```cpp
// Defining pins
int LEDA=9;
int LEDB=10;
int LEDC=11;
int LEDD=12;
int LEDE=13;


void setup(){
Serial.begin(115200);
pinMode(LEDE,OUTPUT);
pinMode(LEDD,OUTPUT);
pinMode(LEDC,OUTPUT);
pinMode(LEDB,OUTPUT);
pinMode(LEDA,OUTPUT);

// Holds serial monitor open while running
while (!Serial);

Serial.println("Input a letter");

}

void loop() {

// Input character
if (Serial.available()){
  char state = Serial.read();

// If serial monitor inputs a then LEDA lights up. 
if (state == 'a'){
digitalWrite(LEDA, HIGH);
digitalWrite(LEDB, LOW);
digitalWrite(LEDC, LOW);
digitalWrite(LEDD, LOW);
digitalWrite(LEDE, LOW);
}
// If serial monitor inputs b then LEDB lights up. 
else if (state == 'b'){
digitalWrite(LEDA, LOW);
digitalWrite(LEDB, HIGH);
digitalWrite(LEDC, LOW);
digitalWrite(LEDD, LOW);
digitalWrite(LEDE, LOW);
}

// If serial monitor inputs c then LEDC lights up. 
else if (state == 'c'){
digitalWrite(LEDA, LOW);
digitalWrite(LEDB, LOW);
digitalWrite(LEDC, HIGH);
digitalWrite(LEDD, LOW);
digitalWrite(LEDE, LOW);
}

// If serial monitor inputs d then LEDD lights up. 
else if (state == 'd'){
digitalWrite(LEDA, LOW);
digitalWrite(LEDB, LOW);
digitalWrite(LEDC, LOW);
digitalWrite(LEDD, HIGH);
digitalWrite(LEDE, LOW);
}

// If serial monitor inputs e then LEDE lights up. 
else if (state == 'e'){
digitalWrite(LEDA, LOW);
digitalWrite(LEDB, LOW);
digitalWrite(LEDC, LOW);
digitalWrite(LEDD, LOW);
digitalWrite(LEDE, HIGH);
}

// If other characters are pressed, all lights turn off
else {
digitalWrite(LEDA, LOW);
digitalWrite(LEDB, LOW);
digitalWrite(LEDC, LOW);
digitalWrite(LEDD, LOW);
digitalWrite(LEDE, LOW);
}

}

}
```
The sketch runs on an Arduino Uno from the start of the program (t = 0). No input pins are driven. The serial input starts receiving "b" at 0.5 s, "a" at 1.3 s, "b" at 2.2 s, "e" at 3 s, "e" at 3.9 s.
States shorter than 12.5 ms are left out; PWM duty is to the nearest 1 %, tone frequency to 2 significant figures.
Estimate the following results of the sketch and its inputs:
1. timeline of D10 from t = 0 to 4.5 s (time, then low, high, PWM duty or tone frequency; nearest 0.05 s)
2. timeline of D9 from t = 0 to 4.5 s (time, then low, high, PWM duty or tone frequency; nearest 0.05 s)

0 s low; 0.5 s high; 1.3 s low; 2.2 s high; 3 s low
0 s low; 1.3 s high; 2.2 s low
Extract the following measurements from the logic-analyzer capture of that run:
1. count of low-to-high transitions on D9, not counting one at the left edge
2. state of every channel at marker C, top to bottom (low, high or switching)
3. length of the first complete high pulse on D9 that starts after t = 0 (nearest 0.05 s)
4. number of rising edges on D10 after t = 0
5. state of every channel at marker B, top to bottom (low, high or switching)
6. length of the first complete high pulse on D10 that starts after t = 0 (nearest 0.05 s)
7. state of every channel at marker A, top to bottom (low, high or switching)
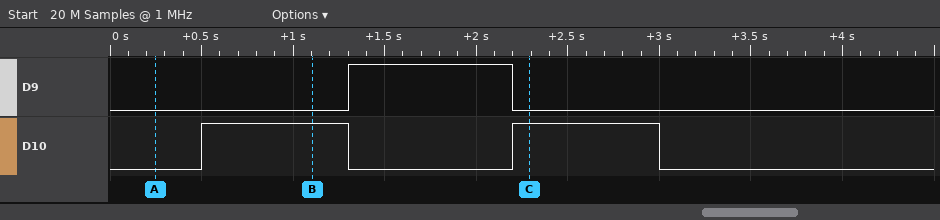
1
D9 low, D10 high
0.90 s
2
D9 low, D10 high
0.80 s
D9 low, D10 low
